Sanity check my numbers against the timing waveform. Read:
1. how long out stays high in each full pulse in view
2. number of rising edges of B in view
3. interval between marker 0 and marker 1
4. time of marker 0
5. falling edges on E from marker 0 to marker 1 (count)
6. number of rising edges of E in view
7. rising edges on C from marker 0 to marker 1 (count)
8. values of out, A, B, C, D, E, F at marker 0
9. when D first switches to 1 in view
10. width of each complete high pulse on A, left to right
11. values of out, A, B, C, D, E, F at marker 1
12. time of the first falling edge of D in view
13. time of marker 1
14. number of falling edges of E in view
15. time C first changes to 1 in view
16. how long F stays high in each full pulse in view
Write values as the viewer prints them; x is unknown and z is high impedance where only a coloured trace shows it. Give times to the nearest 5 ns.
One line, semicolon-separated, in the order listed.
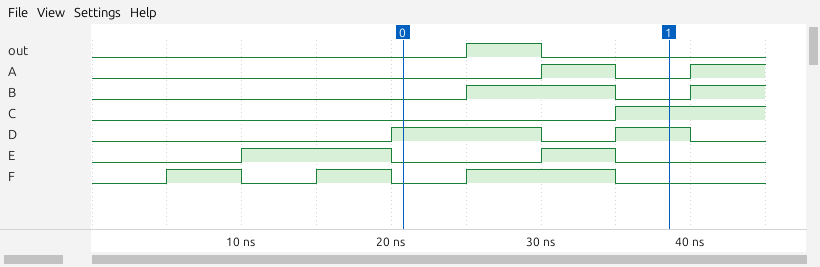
5 ns; 2; 20 ns; 20 ns; 1; 2; 1; out=0, A=0, B=0, C=0, D=1, E=0, F=0; 20 ns; 5 ns; out=0, A=0, B=0, C=1, D=1, E=0, F=0; 30 ns; 40 ns; 2; 35 ns; 5 ns, 5 ns, 10 ns
